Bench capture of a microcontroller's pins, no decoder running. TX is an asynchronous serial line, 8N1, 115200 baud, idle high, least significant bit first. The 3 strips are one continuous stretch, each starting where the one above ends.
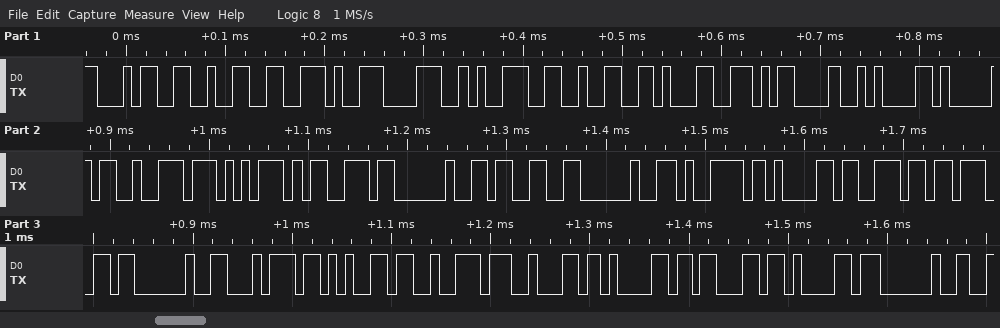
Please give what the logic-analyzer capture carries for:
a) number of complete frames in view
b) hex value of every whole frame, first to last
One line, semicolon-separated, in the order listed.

29; 34 32 2E 38 39 32 31 0D 0A 41 72 75 73 20 33 20 79 61 6E 67 20 74 65 72 62 61 63 61 20
